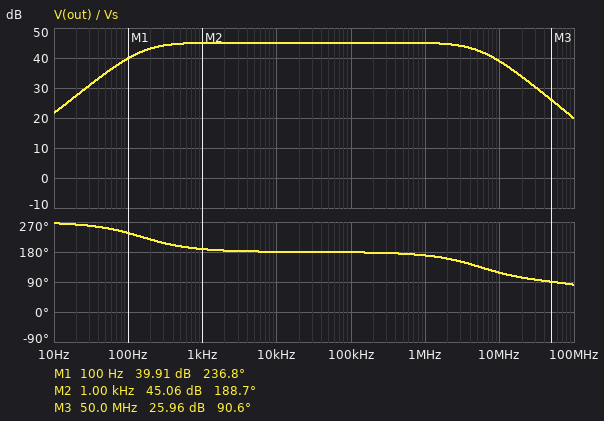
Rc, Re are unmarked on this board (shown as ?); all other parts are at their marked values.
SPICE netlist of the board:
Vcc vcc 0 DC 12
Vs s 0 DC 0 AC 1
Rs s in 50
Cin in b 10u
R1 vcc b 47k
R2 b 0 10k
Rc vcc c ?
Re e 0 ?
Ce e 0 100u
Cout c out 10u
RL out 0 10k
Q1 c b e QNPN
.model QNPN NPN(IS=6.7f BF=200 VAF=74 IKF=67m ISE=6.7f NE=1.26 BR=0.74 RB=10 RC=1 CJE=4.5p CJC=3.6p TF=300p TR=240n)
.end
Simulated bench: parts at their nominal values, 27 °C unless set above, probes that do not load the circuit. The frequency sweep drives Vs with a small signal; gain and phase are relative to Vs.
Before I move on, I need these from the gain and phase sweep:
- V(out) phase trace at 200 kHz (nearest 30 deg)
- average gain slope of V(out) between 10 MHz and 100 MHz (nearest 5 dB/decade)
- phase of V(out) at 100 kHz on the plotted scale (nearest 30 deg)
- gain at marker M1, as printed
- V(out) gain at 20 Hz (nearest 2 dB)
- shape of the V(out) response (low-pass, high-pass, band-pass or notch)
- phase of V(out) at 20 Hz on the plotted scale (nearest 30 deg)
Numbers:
180 deg
-20 dB/decade
180 deg
39.91 dB
28 dB
band-pass
270 deg
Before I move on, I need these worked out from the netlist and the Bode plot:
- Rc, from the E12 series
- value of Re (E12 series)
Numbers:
2.7 kΩ
470 Ω
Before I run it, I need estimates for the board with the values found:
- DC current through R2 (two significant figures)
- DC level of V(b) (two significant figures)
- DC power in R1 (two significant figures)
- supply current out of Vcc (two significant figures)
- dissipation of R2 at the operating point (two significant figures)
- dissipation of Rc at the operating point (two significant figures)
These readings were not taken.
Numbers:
190 µA
1.9 V
2.2 mW
2.8 mA
370 µW
18 mW
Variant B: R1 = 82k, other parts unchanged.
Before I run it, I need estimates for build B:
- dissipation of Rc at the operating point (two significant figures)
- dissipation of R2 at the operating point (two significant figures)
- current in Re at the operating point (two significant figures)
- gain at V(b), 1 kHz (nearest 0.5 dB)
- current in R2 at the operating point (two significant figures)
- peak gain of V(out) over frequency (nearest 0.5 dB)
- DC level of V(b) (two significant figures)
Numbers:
3.6 mW
150 µW
1.2 mA
0 dB
120 µA
39.0 dB
1.2 V
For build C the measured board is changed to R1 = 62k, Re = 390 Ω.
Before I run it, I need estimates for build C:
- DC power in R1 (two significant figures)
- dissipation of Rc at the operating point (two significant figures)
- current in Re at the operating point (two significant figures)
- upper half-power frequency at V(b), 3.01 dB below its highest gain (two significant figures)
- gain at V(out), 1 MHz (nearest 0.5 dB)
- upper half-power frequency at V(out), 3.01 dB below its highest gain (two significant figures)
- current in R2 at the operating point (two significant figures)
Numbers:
1.8 mW
12 mW
2.1 mA
8.0 MHz
43.5 dB
7.2 MHz
150 µA
